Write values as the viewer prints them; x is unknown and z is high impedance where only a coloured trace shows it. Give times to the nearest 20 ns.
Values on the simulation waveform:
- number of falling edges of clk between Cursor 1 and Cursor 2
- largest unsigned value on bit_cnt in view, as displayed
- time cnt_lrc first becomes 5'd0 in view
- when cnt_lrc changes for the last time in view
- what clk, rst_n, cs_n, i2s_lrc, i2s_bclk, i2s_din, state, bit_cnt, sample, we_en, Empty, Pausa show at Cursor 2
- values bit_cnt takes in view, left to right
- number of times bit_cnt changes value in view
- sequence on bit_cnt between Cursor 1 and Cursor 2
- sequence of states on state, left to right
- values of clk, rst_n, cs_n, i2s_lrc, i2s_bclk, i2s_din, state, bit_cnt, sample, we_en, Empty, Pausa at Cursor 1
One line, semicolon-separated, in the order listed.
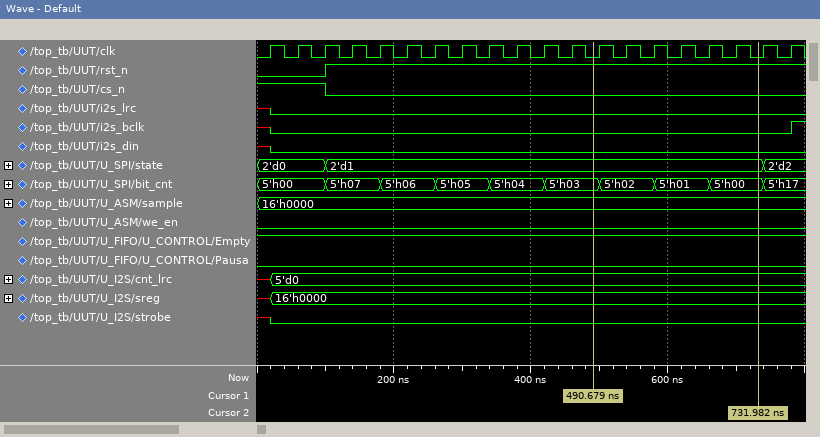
6; 5'h17; 20 ns; 20 ns; clk=0, rst_n=1, cs_n=0, i2s_lrc=0, i2s_bclk=0, i2s_din=0, state=2'd1, bit_cnt=5'h00, sample=16'h0000, we_en=0, Empty=1, Pausa=0; 5'h00, 5'h07, 5'h06, 5'h05, 5'h04, 5'h03, 5'h02, 5'h01, 5'h00, 5'h17; 9; 5'h03, 5'h02, 5'h01, 5'h00; 2'd0, 2'd1, 2'd2; clk=0, rst_n=1, cs_n=0, i2s_lrc=0, i2s_bclk=0, i2s_din=0, state=2'd1, bit_cnt=5'h03, sample=16'h0000, we_en=0, Empty=1, Pausa=0
